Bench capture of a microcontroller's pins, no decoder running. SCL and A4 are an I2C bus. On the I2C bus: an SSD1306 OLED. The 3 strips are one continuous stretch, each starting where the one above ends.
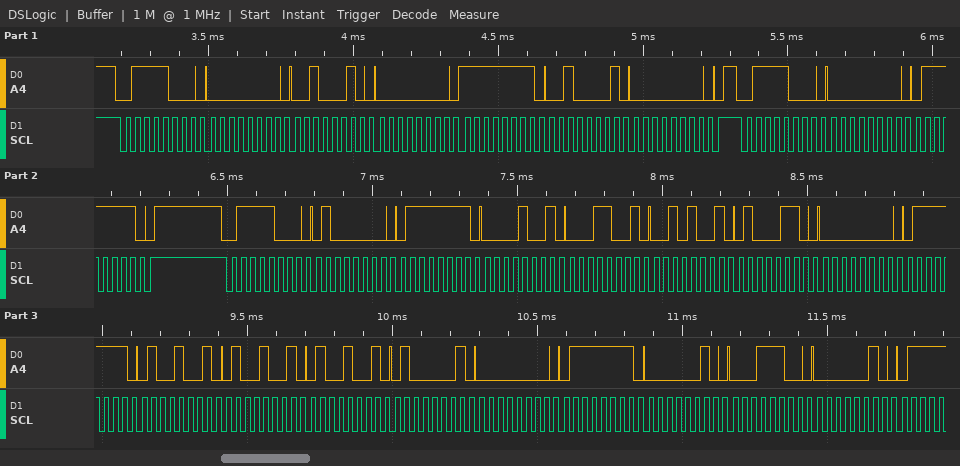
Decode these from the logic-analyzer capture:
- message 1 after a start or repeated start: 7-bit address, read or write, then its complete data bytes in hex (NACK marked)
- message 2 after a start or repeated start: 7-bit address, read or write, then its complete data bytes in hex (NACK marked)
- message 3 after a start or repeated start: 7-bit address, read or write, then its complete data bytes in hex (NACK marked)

0x3C write: 00 22 00 FF 21 00
0x3C write: 00 7F
0x3C write: 40 7F 09 19 29 46 00 7F 49 49 49 41 00 7F 02 1C 02
